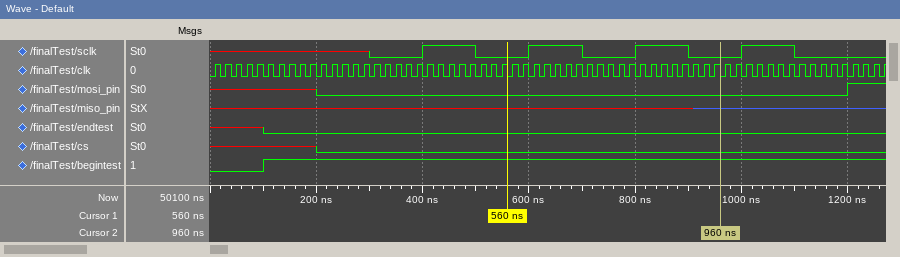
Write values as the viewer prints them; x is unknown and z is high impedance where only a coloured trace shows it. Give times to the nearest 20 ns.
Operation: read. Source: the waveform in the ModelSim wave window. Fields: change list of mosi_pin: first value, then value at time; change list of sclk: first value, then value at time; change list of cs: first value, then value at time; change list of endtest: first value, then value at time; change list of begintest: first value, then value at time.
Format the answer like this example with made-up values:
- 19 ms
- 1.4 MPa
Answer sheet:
- x, 0 at 200 ns, 1 at 1200 ns
- x, 0 at 300 ns, 1 at 400 ns, 0 at 500 ns, 1 at 600 ns, 0 at 700 ns, 1 at 800 ns, 0 at 900 ns, 1 at 1000 ns, 0 at 1100 ns
- x, 0 at 200 ns
- x, 0 at 100 ns
- 0, 1 at 100 ns
